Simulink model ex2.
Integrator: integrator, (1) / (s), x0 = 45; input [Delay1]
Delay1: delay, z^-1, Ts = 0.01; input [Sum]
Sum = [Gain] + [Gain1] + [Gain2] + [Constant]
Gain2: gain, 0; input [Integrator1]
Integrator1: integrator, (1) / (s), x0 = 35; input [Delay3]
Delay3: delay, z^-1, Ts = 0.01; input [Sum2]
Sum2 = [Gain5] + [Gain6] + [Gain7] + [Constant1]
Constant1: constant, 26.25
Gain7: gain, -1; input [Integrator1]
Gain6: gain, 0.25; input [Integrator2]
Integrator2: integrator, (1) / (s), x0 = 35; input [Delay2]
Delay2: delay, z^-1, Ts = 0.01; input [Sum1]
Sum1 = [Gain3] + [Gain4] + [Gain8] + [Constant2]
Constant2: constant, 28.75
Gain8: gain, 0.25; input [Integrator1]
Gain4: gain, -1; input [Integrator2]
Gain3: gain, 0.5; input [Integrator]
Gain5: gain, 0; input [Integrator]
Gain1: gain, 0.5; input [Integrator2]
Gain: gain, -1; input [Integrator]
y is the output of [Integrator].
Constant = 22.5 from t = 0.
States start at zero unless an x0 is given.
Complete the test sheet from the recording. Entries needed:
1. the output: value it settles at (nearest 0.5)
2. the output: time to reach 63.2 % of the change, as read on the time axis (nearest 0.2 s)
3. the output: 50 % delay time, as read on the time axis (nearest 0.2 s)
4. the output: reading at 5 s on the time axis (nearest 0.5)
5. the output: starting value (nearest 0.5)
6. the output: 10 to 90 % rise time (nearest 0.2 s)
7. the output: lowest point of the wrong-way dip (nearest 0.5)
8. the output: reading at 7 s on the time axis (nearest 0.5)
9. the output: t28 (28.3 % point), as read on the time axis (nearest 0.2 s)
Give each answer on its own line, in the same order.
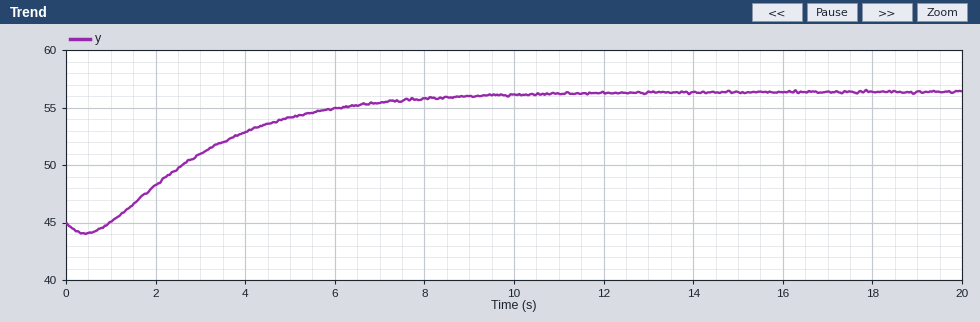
56.5
3.6 s
2.8 s
54.0
45.0
5.2 s
44.0
55.5
2.0 s
